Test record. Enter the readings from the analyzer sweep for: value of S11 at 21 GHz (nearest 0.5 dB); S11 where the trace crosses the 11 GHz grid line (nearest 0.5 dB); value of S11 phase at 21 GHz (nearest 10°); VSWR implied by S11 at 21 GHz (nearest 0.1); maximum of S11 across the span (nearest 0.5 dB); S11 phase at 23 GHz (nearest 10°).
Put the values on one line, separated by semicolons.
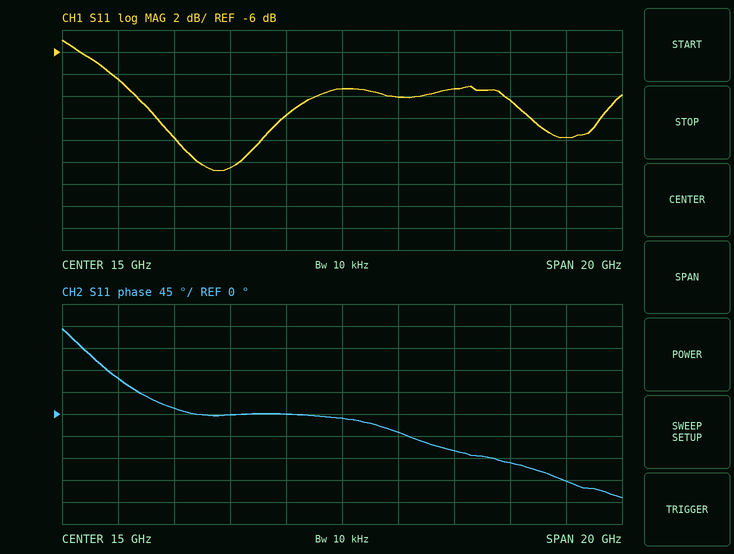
-10.5 dB; -16.5 dB; -100°; 1.9; -5.0 dB; -140°
